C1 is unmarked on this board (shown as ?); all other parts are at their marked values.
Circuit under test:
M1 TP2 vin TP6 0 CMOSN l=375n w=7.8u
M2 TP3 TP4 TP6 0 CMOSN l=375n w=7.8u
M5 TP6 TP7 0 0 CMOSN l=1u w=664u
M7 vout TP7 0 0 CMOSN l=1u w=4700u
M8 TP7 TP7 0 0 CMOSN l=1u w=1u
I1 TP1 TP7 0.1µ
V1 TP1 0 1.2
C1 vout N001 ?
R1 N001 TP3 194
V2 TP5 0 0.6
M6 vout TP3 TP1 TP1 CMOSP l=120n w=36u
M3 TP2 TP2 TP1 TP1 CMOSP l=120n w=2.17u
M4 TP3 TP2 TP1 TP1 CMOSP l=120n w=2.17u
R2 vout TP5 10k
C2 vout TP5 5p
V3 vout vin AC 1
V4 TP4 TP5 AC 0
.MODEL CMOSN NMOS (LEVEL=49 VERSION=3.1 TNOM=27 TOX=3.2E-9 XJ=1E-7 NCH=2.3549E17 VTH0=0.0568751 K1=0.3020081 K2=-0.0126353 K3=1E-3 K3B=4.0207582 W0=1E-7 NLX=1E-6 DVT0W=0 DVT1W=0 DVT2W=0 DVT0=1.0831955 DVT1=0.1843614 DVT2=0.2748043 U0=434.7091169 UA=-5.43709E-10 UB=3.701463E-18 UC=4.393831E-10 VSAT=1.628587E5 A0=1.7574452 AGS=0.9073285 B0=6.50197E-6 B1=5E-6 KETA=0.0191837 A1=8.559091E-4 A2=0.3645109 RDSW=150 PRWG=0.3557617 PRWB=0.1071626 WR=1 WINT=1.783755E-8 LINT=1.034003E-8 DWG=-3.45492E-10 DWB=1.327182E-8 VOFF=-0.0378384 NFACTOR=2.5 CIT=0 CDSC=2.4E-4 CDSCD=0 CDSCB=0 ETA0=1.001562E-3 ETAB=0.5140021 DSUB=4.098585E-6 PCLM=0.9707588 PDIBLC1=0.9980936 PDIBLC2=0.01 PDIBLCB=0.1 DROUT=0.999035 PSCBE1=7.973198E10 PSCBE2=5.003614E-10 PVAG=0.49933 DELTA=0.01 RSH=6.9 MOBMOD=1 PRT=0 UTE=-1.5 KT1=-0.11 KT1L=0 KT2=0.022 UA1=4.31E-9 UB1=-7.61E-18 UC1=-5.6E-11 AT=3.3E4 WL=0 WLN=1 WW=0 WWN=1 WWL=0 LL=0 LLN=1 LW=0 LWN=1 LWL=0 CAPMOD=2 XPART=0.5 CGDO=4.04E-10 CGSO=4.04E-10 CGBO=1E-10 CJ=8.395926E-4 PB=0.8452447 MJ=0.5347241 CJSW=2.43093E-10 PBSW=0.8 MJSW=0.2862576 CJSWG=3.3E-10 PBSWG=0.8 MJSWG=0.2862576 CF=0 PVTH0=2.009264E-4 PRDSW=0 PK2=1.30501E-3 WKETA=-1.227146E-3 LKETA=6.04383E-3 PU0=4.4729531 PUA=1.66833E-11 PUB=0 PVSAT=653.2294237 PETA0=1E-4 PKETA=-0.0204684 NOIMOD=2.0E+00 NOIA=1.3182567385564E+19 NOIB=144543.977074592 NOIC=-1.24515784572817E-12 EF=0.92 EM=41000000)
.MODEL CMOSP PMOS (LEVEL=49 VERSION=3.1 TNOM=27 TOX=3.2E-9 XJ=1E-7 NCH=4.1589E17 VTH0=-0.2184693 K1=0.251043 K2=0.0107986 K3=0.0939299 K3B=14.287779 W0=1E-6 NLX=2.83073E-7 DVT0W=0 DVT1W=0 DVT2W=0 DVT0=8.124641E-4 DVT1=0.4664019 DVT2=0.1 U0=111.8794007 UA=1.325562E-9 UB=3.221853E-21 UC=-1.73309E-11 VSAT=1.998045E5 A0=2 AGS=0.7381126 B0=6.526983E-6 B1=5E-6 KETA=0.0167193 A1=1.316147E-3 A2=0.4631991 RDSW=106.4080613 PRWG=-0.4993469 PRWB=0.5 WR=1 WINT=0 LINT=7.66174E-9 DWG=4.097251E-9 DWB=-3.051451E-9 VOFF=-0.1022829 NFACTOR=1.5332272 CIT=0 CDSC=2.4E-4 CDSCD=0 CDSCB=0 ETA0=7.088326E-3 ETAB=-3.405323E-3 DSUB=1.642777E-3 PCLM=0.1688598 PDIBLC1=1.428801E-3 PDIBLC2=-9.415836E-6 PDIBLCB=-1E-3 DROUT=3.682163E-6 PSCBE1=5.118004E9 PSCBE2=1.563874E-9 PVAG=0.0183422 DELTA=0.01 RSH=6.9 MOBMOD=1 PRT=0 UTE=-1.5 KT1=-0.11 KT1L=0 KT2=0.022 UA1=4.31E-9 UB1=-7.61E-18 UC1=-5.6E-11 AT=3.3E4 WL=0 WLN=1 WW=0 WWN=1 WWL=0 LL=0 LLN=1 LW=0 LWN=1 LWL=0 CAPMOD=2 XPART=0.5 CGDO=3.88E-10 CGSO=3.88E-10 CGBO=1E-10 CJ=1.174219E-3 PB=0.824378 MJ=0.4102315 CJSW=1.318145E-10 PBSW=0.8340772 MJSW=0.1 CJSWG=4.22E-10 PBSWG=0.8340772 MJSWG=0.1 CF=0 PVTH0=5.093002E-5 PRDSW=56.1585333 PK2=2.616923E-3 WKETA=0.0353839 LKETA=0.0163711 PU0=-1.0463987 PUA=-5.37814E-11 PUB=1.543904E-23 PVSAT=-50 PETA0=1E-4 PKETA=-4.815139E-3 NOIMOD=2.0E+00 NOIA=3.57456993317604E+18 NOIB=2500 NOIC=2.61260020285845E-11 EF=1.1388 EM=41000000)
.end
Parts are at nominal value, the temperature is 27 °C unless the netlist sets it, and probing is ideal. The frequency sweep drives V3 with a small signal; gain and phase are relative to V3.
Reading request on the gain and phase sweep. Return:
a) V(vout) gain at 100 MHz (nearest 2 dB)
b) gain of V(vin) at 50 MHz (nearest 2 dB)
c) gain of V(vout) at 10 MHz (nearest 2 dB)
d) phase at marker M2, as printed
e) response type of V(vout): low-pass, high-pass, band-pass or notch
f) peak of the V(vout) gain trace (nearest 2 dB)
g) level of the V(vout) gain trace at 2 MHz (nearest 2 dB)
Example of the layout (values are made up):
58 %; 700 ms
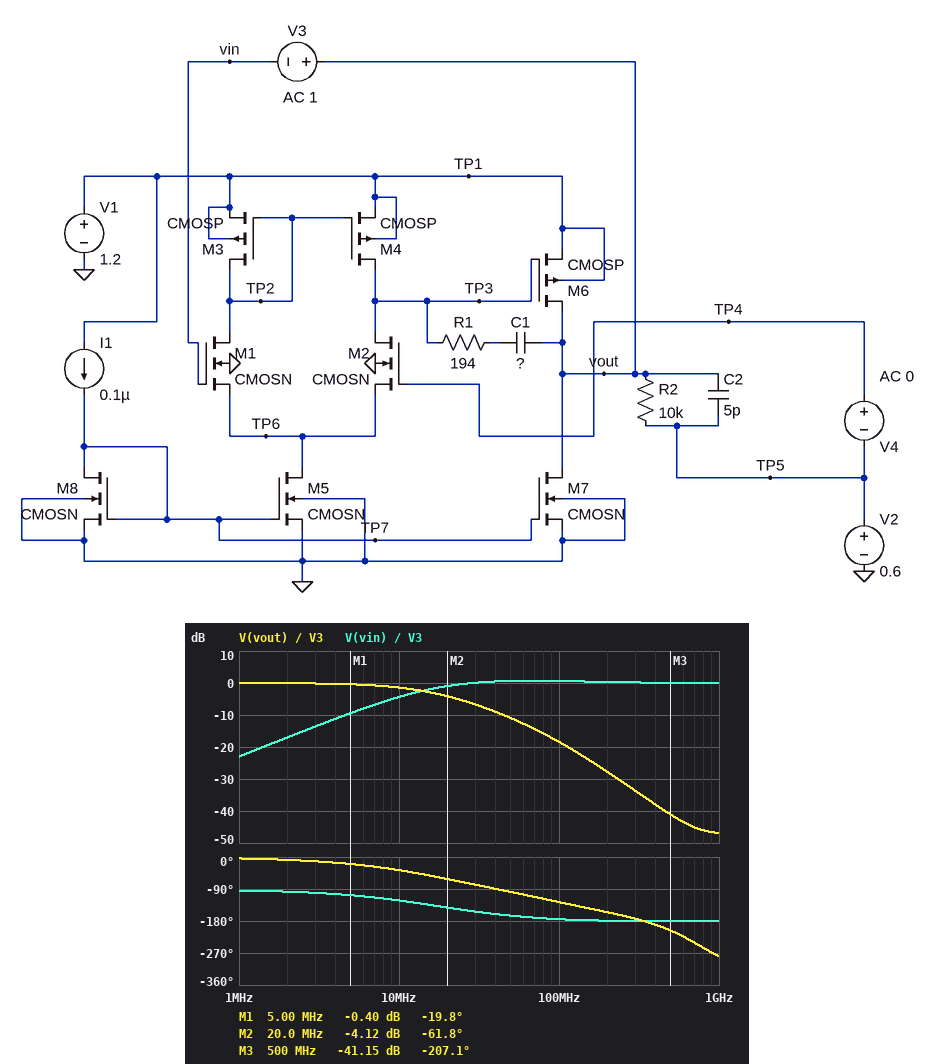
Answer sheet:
-18 dB; 0 dB; -2 dB; -61.8 deg; low-pass; 0 dB; 0 dB
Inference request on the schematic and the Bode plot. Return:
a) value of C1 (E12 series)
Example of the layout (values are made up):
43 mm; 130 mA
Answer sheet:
6.8 pF
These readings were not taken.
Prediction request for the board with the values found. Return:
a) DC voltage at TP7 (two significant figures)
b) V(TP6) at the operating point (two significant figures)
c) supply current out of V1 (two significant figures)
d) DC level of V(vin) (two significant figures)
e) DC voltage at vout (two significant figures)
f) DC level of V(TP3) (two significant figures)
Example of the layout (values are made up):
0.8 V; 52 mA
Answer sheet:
190 mV; 190 mV; 610 µA; 600 mV; 600 mV; 590 mV
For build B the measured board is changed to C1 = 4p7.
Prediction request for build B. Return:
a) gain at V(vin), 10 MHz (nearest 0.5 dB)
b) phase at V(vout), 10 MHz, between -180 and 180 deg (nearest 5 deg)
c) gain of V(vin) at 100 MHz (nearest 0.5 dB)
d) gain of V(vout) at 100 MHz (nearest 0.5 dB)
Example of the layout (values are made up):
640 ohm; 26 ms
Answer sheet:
-7.0 dB; -25 deg; 1.0 dB; -15.0 dB
